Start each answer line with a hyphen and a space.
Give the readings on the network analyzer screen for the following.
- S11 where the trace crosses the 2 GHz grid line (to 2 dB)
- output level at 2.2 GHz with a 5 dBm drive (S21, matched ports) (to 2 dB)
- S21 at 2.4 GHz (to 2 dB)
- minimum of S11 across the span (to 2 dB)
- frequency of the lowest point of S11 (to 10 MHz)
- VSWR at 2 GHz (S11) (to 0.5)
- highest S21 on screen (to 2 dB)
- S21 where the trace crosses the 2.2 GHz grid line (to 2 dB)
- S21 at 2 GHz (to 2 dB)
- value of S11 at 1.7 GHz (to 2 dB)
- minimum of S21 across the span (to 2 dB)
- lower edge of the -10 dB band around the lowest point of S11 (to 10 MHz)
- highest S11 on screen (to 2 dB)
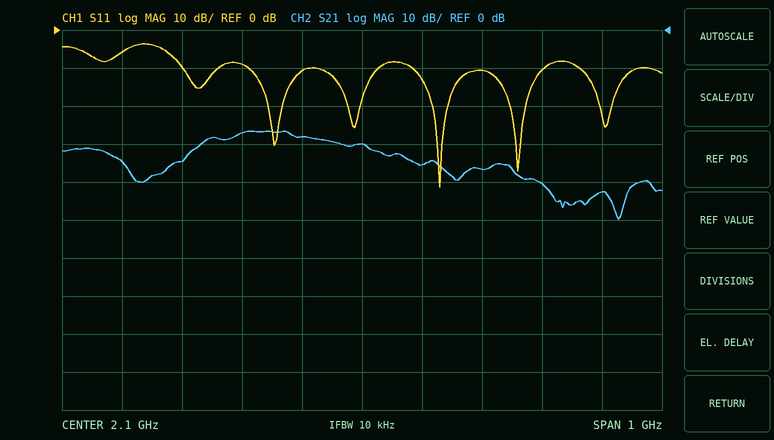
- -10 dB
- -30 dBm
- -40 dB
- -42 dB
- 2.23 GHz
- 2.0
- -26 dB
- -36 dB
- -28 dB
- -6 dB
- -50 dB
- 2.18 GHz
- -4 dB
